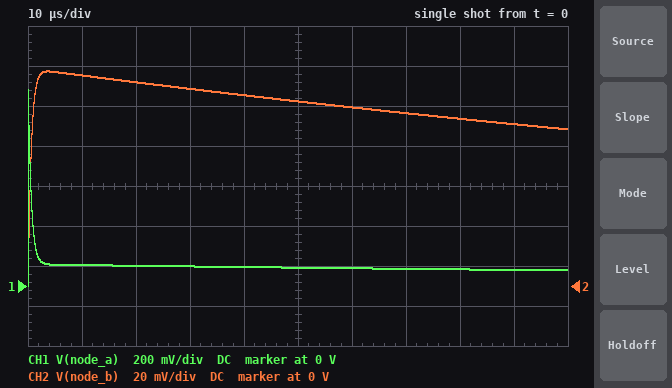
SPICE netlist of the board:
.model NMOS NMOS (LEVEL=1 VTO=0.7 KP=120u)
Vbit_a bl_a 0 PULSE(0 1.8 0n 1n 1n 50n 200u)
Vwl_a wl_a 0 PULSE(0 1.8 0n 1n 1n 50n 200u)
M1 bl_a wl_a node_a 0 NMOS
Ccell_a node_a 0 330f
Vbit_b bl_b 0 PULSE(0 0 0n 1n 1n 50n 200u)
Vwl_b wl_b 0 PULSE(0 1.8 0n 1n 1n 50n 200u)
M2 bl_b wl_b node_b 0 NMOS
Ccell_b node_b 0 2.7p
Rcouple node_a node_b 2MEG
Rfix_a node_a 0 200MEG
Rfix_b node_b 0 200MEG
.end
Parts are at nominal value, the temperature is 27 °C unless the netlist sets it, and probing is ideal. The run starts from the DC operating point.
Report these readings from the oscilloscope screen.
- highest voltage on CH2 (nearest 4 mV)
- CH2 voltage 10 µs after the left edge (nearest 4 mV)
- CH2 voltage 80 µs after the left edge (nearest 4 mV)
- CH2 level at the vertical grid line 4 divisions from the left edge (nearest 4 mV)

108 mV
104 mV
84 mV
96 mV
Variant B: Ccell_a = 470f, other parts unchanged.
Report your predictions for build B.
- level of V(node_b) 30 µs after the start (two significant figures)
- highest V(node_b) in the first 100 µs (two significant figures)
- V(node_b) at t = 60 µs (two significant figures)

130 mV
140 mV
120 mV
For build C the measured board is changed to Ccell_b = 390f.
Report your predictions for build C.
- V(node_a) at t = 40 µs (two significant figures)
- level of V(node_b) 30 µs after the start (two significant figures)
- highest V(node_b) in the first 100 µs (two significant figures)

260 mV
300 mV
440 mV
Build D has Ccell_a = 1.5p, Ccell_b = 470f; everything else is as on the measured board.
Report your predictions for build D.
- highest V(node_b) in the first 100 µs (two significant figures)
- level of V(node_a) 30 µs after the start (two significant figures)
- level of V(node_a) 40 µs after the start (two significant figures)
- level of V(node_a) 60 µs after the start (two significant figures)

560 mV
500 mV
470 mV
430 mV
